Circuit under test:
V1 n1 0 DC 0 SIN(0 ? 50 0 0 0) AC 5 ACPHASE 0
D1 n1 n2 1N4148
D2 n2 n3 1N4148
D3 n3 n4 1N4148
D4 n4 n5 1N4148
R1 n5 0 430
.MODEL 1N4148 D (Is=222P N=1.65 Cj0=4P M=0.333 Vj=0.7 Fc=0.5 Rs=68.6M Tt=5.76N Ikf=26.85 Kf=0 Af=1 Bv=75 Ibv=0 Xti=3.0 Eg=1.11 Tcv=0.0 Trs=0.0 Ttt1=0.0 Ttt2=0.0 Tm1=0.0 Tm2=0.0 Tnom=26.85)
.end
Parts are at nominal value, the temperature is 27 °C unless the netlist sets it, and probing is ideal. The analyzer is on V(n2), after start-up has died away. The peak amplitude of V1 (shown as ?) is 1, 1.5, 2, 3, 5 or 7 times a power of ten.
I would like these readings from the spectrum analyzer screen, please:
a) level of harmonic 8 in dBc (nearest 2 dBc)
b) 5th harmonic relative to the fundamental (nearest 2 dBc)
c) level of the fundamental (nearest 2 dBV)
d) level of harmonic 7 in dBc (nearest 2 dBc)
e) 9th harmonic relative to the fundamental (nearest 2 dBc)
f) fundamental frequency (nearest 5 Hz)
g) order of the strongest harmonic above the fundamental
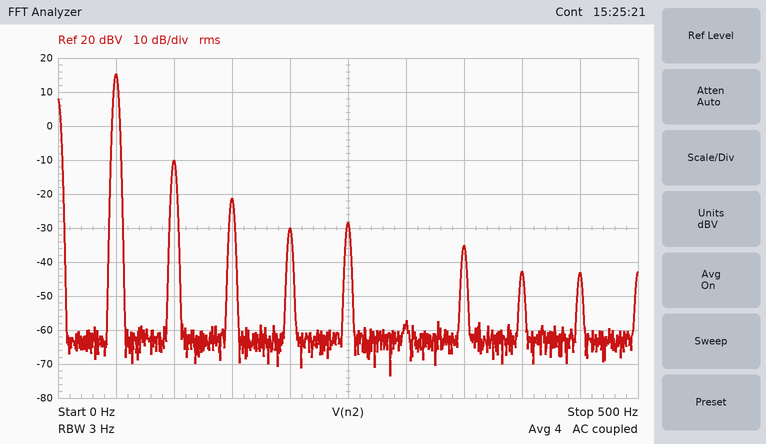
-58 dBc
-44 dBc
16 dBV
-50 dBc
-58 dBc
50 Hz
2
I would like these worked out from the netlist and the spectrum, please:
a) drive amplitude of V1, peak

10 V
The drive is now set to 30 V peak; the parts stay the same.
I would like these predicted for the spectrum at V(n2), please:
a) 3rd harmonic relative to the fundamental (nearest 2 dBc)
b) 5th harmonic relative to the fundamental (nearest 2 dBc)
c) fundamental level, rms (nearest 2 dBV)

-44 dBc
-50 dBc
26 dBV
